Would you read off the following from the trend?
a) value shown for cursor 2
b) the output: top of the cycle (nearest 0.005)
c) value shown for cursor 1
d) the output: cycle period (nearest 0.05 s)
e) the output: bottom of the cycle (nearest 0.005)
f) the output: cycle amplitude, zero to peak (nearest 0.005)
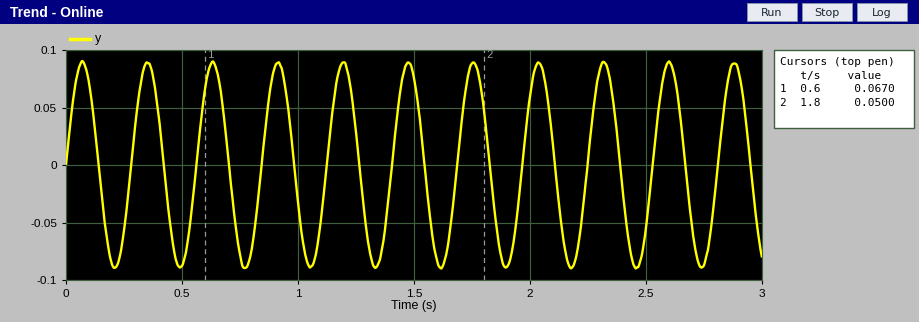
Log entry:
0.0500
0.090
0.0670
0.30 s
-0.090
0.090
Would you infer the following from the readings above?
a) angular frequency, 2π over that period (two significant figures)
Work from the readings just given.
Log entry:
21 rad/s
